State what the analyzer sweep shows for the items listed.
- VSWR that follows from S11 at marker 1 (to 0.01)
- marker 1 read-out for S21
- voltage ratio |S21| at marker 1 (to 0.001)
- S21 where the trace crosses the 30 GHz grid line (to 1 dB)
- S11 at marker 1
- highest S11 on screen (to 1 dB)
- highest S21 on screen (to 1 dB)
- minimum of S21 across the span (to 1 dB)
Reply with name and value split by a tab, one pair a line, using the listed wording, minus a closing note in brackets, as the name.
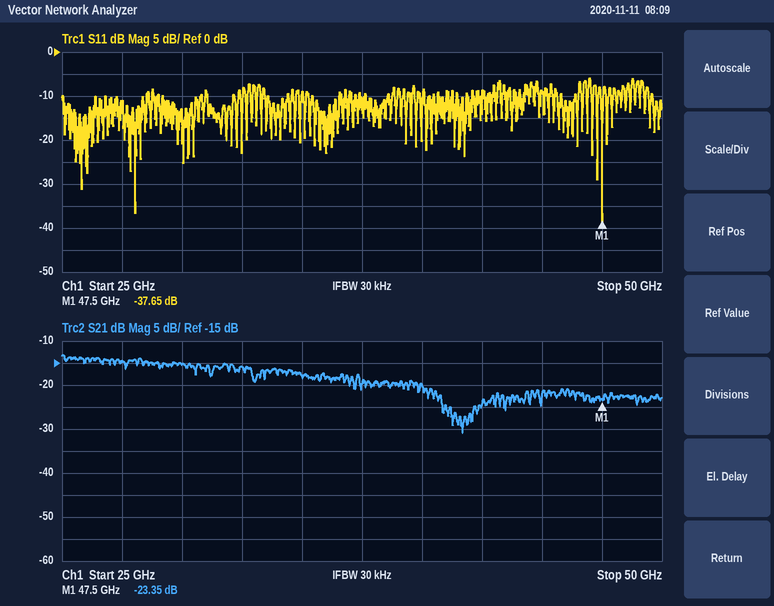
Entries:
VSWR that follows from S11 at marker 1	1.03
marker 1 read-out for S21	-23.35 dB
voltage ratio |S21| at marker 1	0.068
S21 where the trace crosses the 30 GHz grid line	-15 dB
S11 at marker 1	-37.65 dB
highest S11 on screen	-6 dB
highest S21 on screen	-13 dB
minimum of S21 across the span	-31 dB
